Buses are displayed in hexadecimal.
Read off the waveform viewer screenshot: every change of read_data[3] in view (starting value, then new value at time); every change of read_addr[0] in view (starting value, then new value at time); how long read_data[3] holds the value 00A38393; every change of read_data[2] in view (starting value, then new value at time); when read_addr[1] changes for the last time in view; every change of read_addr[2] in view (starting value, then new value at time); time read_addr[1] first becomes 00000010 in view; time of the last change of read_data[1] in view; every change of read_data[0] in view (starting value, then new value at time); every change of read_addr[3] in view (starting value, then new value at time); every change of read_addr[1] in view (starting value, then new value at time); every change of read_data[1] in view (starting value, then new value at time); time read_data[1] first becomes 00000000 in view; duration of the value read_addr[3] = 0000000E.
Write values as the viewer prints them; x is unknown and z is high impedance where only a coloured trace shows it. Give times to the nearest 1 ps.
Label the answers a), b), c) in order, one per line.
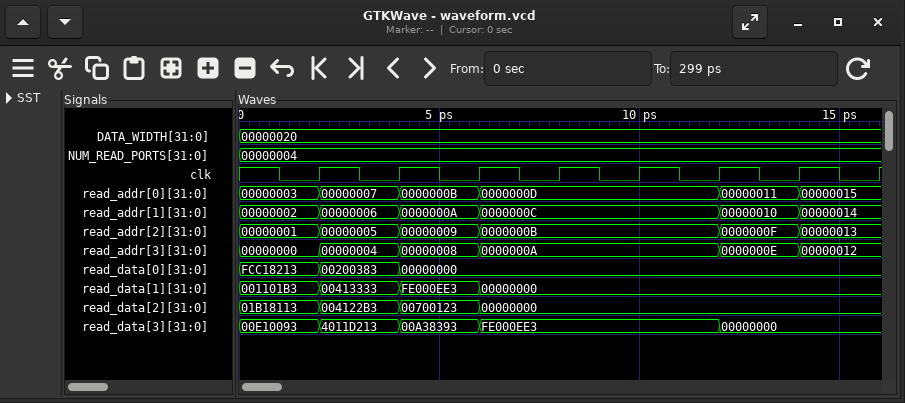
a) 00E10093, 4011D213 at 2 ps, 00A38393 at 4 ps, FE000EE3 at 6 ps, 00000000 at 12 ps
b) 00000003, 00000007 at 2 ps, 0000000B at 4 ps, 0000000D at 6 ps, 00000011 at 12 ps, 00000015 at 14 ps
c) 2 ps
d) 01B18113, 004122B3 at 2 ps, 00700123 at 4 ps, 00000000 at 6 ps
e) 14 ps
f) 00000001, 00000005 at 2 ps, 00000009 at 4 ps, 0000000B at 6 ps, 0000000F at 12 ps, 00000013 at 14 ps
g) 12 ps
h) 6 ps
i) FCC18213, 00200383 at 2 ps, 00000000 at 4 ps
j) 00000000, 00000004 at 2 ps, 00000008 at 4 ps, 0000000A at 6 ps, 0000000E at 12 ps, 00000012 at 14 ps
k) 00000002, 00000006 at 2 ps, 0000000A at 4 ps, 0000000C at 6 ps, 00000010 at 12 ps, 00000014 at 14 ps
l) 001101B3, 00413333 at 2 ps, FE000EE3 at 4 ps, 00000000 at 6 ps
m) 6 ps
n) 2 ps
